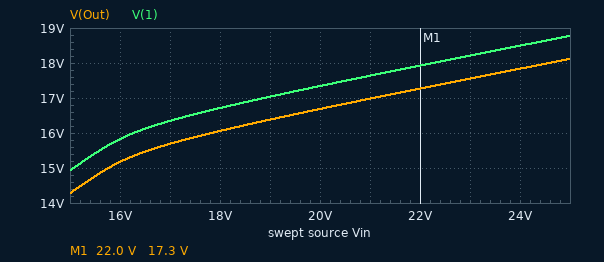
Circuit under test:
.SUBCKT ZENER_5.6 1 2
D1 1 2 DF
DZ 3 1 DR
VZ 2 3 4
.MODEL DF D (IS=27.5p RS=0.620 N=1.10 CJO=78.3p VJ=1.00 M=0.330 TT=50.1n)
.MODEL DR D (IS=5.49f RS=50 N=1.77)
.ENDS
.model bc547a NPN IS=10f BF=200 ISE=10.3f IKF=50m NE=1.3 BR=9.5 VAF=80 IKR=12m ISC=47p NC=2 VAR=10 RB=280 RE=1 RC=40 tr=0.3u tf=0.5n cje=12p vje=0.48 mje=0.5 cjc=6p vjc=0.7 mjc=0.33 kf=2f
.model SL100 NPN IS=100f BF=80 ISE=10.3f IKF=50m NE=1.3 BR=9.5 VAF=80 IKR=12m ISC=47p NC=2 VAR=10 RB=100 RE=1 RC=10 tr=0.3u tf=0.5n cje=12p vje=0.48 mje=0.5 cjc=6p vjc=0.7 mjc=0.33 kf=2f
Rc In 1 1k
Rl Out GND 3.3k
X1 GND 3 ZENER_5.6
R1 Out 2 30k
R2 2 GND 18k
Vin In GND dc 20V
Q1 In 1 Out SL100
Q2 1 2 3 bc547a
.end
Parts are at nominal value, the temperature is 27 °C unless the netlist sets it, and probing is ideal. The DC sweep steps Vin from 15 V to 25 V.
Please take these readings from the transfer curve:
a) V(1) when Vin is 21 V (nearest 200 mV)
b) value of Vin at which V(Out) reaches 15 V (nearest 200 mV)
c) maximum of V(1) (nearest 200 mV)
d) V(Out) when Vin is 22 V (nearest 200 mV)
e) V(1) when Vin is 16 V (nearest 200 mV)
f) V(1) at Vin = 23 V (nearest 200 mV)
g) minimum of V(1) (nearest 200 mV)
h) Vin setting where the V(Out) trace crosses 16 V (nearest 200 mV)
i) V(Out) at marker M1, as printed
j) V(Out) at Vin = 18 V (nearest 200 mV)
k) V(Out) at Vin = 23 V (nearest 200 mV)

17.6 V
15.8 V
18.8 V
17.2 V
15.8 V
18.2 V
15.0 V
17.8 V
17.3 V
16.0 V
17.6 V
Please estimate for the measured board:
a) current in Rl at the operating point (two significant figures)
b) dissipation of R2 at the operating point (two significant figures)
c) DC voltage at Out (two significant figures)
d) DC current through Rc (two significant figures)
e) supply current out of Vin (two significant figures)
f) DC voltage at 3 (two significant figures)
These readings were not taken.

5.1 mA
2.0 mW
17 V
2.7 mA
8.0 mA
5.4 V
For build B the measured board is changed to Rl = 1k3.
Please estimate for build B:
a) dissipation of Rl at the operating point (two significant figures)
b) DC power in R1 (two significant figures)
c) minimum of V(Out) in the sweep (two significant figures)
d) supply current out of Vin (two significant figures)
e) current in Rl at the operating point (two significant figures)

210 mW
3.7 mW
14 V
16 mA
13 mA
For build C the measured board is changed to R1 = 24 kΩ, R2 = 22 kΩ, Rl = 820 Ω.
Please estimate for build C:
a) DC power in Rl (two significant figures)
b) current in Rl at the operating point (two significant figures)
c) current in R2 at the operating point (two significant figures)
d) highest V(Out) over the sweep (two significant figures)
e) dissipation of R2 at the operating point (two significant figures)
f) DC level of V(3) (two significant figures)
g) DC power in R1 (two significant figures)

240 mW
17 mA
280 µA
15 V
1.8 mW
5.5 V
2.5 mW
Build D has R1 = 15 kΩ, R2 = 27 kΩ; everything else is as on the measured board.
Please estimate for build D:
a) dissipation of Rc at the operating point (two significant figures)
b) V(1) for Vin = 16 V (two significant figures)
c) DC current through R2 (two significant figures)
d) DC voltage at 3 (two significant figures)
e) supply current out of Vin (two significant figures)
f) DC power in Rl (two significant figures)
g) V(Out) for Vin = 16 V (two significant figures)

70 mW
11 V
240 µA
5.7 V
12 mA
37 mW
10 V
